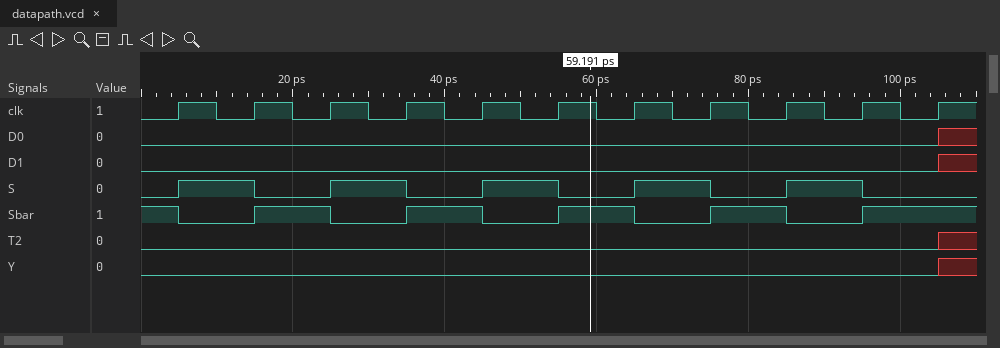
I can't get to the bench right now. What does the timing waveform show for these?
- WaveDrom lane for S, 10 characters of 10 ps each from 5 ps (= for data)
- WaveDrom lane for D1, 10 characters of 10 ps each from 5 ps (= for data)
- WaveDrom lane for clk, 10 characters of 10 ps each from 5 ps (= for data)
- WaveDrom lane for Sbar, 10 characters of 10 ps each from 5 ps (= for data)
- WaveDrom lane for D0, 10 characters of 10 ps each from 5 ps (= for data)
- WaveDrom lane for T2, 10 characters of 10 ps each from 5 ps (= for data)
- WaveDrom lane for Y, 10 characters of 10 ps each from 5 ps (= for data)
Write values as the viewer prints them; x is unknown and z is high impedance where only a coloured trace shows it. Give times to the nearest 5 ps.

{name: 'S', wave: '1010101010'}
{name: 'D1', wave: '0.........'}
{name: 'clk', wave: 'p.........'}
{name: 'Sbar', wave: '0101010101'}
{name: 'D0', wave: '0.........'}
{name: 'T2', wave: '0.........'}
{name: 'Y', wave: '0.........'}
